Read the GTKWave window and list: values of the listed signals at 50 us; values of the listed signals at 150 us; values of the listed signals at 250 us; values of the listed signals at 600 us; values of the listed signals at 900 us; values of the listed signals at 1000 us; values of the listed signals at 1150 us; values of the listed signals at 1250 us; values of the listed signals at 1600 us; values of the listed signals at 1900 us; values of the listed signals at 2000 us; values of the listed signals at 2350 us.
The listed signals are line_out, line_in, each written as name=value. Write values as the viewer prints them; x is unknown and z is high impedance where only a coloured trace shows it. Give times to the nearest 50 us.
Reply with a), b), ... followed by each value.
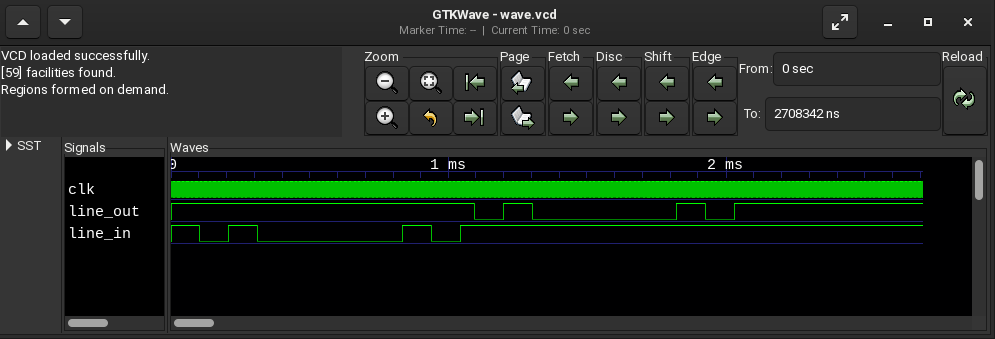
a) line_out=1, line_in=1
b) line_out=1, line_in=0
c) line_out=1, line_in=1
d) line_out=1, line_in=0
e) line_out=1, line_in=1
f) line_out=1, line_in=0
g) line_out=0, line_in=1
h) line_out=1, line_in=1
i) line_out=0, line_in=1
j) line_out=1, line_in=1
k) line_out=0, line_in=1
l) line_out=1, line_in=1
